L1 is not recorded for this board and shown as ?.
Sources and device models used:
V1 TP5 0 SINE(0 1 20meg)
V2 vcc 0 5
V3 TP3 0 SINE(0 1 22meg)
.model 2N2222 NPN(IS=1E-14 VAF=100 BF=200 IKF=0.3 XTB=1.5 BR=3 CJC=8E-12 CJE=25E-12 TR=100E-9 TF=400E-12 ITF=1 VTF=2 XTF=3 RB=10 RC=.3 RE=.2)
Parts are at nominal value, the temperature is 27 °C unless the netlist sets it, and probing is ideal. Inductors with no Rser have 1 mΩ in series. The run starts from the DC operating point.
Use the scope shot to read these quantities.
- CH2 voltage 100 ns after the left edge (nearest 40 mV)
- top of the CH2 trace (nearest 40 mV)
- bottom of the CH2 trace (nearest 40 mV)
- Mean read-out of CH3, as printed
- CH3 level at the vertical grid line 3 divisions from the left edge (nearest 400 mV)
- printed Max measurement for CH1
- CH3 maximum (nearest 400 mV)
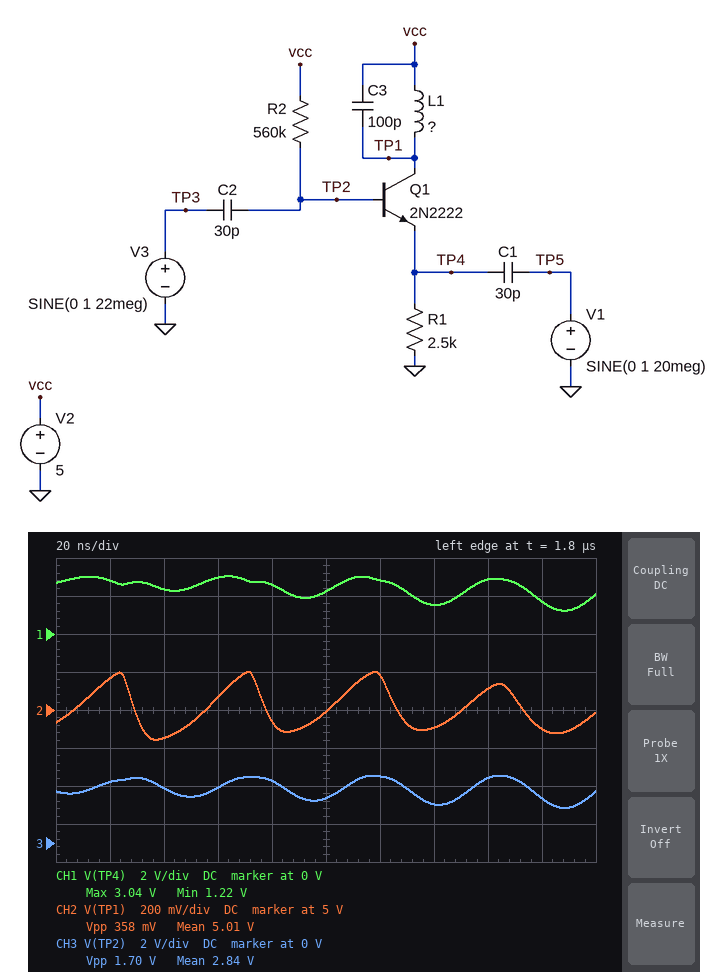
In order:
5.00 V
5.20 V
4.84 V
2.84 V
2.8 V
3.04 V
3.6 V
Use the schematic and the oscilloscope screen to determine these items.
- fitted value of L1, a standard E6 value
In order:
4.7 µH
